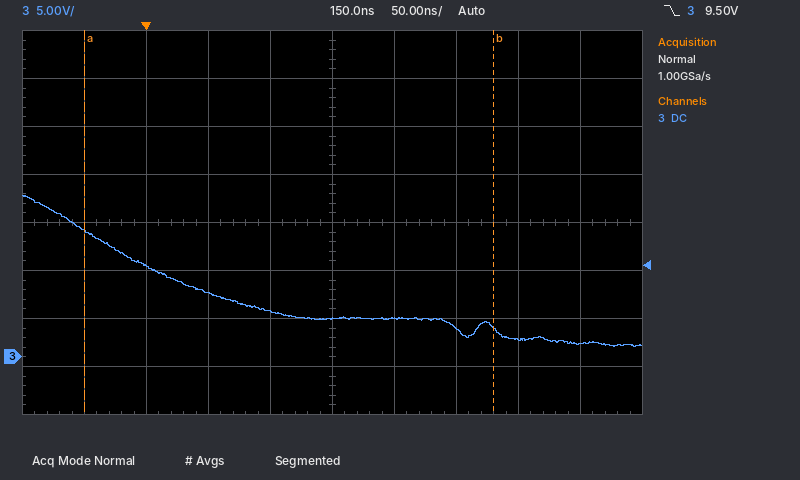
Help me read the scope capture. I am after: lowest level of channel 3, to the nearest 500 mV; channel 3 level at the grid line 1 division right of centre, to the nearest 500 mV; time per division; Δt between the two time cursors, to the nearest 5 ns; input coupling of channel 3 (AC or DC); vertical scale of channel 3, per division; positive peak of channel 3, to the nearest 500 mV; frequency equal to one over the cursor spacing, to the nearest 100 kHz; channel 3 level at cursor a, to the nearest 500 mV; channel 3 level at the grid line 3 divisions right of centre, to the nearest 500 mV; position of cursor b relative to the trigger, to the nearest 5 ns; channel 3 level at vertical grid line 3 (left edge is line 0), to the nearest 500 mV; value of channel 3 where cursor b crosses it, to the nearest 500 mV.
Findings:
1.0 V
4.0 V
50 ns
330 ns
DC
5 V
17.0 V
3.0 MHz
13.0 V
2.0 V
+280 ns
6.5 V
3.0 V
